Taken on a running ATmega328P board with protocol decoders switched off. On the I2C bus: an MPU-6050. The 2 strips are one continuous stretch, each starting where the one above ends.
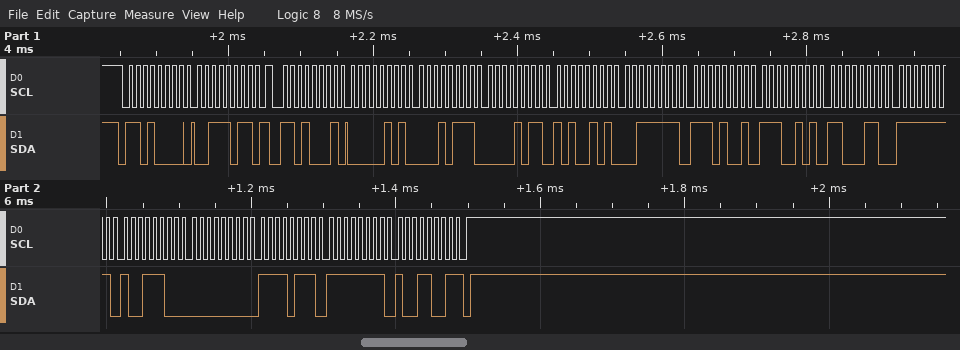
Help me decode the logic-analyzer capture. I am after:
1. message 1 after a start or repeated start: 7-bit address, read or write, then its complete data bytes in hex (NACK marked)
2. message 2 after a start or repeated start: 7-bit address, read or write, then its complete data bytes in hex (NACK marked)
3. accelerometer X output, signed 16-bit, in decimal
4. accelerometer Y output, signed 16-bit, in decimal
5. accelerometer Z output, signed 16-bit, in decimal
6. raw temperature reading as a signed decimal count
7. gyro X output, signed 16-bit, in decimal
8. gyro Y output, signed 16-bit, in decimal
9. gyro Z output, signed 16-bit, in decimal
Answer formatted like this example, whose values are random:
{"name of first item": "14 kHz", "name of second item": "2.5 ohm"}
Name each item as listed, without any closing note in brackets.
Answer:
{"message 1 after a start or repeated start: 7-bit address, read or write, then its complete data bytes in hex": "0x68 write: 3B", "message 2 after a start or repeated start: 7-bit address, read or write, then its complete data bytes in hex": "0x68 read: 05 17 0B A5 3F E9 E5 C6 FF 9C 00 F7 FF 99 NACK", "accelerometer X output, signed 16-bit, in decimal": "1303", "accelerometer Y output, signed 16-bit, in decimal": "2981", "accelerometer Z output, signed 16-bit, in decimal": "16361", "raw temperature reading as a signed decimal count": "-6714", "gyro X output, signed 16-bit, in decimal": "-100", "gyro Y output, signed 16-bit, in decimal": "247", "gyro Z output, signed 16-bit, in decimal": "-103"}
